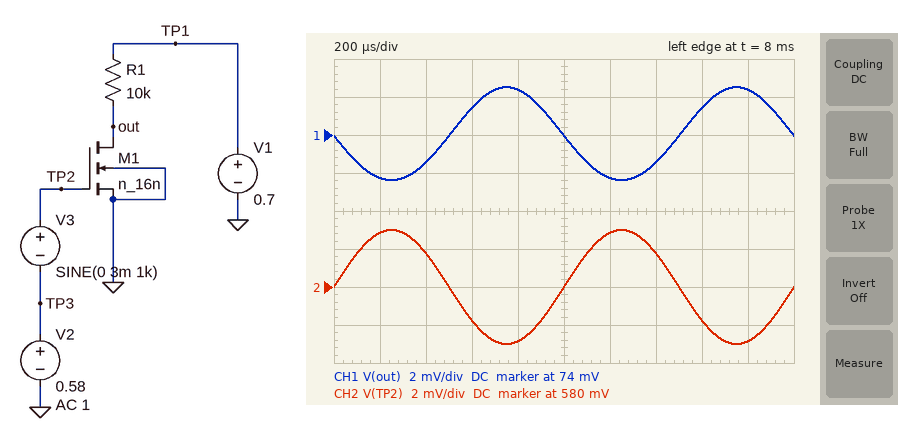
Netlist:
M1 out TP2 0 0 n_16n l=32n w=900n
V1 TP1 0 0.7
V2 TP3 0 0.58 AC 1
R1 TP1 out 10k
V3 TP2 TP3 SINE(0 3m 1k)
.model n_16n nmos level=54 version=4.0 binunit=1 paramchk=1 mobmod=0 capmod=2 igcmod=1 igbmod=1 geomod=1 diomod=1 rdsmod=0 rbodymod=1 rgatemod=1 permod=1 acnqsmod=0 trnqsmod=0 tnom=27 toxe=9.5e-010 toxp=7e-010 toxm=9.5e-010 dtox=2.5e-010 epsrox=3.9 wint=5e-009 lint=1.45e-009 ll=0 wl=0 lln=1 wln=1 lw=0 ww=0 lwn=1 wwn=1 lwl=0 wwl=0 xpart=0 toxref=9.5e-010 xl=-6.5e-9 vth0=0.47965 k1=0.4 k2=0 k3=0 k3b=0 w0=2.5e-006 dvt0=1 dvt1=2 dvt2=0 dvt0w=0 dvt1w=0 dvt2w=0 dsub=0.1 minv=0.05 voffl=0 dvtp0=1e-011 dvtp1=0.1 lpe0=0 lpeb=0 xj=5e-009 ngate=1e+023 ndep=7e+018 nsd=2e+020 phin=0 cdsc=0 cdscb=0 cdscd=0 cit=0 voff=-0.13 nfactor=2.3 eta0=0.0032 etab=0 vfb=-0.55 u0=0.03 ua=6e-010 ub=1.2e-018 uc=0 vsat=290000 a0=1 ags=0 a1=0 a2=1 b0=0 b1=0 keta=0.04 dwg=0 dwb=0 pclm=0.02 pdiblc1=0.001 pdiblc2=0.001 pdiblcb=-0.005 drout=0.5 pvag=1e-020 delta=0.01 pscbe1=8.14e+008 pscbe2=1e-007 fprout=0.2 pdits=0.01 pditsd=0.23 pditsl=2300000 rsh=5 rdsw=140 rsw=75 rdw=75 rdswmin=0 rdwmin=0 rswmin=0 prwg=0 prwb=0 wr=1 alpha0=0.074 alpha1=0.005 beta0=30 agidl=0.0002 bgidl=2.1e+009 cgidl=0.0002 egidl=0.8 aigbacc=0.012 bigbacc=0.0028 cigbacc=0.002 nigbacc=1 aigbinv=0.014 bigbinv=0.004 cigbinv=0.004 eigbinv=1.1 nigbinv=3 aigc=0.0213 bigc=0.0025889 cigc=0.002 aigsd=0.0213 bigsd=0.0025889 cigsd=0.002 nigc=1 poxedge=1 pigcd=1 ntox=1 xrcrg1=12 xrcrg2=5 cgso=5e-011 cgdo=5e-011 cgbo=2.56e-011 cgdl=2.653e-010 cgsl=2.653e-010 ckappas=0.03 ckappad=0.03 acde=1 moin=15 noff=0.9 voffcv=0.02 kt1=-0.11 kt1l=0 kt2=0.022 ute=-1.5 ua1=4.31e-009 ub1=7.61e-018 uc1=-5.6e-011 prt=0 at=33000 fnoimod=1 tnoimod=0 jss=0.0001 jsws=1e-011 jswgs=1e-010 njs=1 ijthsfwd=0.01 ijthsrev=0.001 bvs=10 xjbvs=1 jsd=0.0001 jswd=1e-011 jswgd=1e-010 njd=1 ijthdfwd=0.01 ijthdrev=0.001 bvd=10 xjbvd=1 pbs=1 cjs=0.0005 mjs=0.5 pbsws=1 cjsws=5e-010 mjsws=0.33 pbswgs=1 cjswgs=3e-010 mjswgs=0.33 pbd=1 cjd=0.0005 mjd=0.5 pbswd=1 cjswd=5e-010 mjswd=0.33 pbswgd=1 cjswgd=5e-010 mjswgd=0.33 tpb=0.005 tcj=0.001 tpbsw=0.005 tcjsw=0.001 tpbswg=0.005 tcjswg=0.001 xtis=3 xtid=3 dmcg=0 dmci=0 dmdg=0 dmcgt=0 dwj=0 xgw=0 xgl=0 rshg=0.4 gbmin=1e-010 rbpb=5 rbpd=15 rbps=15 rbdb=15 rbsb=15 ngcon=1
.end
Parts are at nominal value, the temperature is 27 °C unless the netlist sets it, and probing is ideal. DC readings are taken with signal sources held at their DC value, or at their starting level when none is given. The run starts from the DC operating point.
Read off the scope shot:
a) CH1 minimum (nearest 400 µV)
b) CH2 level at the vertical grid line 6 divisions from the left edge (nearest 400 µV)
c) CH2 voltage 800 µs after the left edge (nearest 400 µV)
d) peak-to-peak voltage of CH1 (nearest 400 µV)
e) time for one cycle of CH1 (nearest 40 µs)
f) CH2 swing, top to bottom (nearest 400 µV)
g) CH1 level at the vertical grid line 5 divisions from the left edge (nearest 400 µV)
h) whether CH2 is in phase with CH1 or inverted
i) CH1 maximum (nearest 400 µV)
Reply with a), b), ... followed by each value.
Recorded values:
a) 71.6 mV
b) 582.8 mV
c) 577.2 mV
d) 4.8 mV
e) 1.00 ms
f) 6.0 mV
g) 74.0 mV
h) inverted
i) 76.4 mV
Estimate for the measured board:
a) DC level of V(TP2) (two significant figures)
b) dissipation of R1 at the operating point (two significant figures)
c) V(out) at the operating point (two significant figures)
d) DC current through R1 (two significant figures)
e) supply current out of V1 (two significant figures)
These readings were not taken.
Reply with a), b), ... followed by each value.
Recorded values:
a) 580 mV
b) 39 µW
c) 74 mV
d) 63 µA
e) 63 µA
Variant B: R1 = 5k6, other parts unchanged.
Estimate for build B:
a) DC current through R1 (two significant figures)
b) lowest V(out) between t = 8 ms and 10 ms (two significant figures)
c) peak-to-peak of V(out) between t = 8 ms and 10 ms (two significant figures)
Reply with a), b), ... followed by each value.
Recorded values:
a) 90 µA
b) 180 mV
c) 24 mV
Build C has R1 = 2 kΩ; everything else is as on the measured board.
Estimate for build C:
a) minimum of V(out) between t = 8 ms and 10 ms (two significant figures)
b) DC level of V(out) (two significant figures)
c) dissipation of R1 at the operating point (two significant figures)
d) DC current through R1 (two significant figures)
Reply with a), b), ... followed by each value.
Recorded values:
a) 490 mV
b) 500 mV
c) 21 µW
d) 100 µA
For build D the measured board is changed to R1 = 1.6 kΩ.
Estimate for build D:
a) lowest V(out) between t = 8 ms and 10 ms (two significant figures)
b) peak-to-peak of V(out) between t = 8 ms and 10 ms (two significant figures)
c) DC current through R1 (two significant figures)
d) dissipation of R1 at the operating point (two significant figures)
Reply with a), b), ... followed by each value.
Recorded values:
a) 530 mV
b) 10 mV
c) 100 µA
d) 17 µW
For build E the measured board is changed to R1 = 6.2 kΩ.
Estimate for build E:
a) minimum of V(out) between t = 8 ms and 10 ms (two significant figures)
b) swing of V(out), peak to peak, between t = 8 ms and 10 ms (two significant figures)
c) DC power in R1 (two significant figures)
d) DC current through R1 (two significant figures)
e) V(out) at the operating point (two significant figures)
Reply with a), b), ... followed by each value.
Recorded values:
a) 150 mV
b) 21 mV
c) 47 µW
d) 87 µA
e) 160 mV
